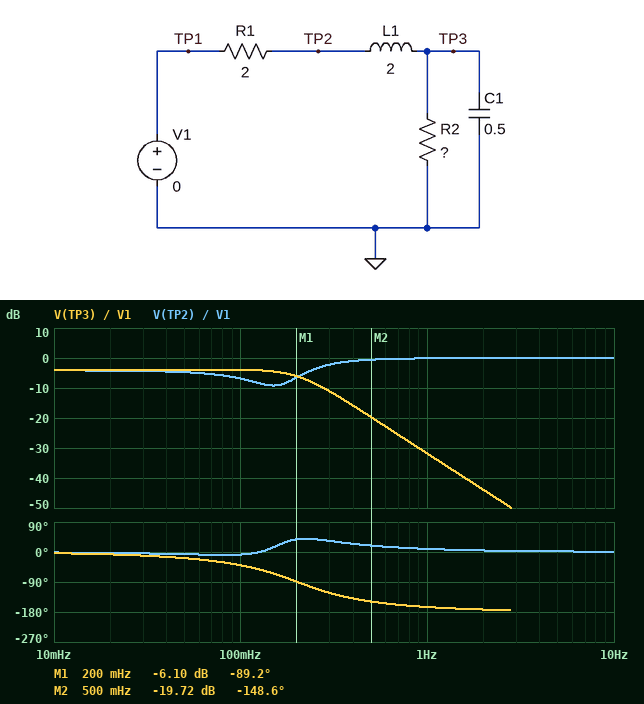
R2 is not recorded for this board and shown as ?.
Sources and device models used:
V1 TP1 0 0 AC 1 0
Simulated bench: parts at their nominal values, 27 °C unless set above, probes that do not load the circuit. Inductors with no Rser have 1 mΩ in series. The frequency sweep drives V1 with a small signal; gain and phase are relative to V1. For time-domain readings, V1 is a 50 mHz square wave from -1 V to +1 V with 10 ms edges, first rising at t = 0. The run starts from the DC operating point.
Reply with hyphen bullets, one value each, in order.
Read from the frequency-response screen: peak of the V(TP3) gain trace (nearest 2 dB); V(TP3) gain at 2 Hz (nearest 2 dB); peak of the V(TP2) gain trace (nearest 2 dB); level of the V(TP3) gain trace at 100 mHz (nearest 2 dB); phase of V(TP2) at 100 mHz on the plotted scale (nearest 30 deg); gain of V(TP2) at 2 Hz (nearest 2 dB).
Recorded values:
- -4 dB
- -44 dB
- 0 dB
- -4 dB
- 0 deg
- 0 dB
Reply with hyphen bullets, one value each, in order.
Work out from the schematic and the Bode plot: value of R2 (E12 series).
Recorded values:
- 3.3 Ω
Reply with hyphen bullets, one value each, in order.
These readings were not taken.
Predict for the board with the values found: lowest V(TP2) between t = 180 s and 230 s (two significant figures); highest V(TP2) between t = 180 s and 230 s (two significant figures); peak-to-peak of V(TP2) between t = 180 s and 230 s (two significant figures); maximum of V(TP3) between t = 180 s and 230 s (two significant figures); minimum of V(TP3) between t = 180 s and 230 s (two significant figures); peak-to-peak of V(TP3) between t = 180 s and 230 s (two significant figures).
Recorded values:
- -1.4 V
- 1.4 V
- 2.7 V
- 720 mV
- -720 mV
- 1.4 V
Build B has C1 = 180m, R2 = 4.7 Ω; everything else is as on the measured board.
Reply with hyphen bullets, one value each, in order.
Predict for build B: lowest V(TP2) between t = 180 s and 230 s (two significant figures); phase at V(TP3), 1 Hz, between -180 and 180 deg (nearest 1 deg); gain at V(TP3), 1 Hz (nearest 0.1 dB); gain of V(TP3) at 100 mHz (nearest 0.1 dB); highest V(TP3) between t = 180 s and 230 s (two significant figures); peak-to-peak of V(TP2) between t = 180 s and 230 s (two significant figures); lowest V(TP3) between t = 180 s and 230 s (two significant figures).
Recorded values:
- -1.3 V
- -159 deg
- -22.7 dB
- -2.8 dB
- 880 mV
- 2.6 V
- -880 mV
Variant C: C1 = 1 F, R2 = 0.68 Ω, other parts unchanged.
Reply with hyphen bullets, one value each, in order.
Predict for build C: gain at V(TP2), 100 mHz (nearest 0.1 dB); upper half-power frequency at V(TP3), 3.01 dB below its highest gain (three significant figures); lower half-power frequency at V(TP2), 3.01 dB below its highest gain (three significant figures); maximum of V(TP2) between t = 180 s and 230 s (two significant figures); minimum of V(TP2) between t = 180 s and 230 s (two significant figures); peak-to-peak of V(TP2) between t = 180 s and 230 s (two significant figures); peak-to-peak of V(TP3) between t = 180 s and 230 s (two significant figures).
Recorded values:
- -7.5 dB
- 172 mHz
- 211 mHz
- 1.7 V
- -1.7 V
- 3.5 V
- 510 mV
